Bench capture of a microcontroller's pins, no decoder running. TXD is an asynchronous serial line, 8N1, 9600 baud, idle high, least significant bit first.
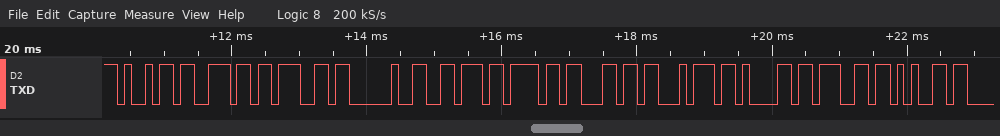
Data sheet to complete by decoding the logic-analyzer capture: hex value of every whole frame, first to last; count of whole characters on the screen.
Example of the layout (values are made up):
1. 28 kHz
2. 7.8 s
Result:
1. 0x69 0x6E 0x67 0x20 0x76 0x6F 0x6C 0x74 0x61 0x67 0x65
2. 11
